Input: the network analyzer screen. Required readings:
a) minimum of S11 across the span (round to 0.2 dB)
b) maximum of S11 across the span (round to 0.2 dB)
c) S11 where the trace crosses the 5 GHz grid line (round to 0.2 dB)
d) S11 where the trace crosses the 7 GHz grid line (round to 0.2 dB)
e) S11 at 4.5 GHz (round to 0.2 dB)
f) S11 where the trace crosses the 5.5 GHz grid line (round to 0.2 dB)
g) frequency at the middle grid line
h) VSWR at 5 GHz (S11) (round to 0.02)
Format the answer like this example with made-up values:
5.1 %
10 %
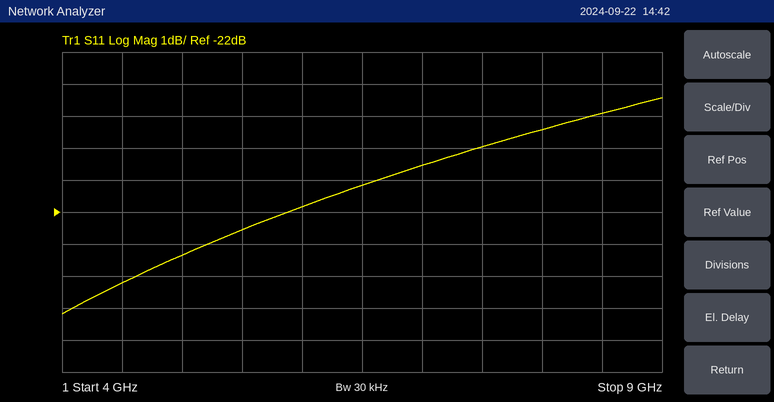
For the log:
-25.2 dB
-18.4 dB
-23.4 dB
-20.6 dB
-24.2 dB
-22.6 dB
6.5 GHz
1.14
